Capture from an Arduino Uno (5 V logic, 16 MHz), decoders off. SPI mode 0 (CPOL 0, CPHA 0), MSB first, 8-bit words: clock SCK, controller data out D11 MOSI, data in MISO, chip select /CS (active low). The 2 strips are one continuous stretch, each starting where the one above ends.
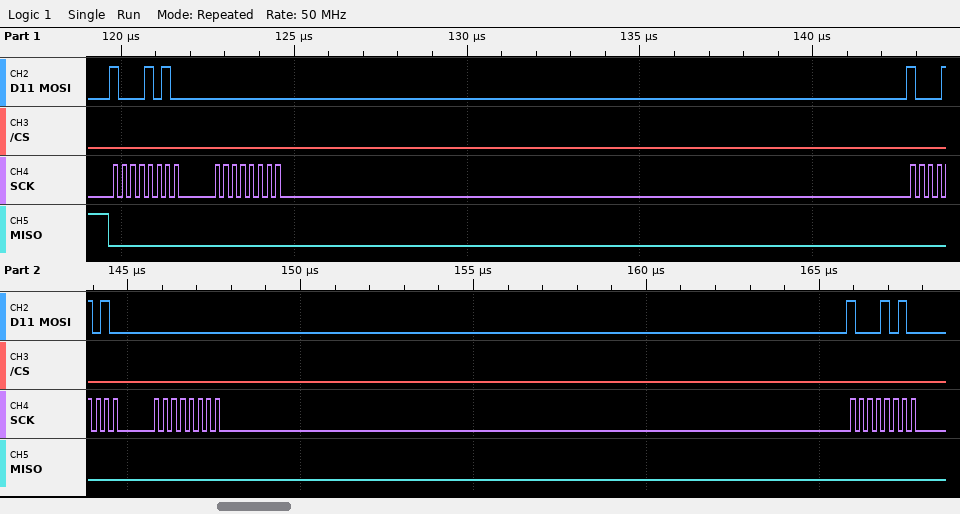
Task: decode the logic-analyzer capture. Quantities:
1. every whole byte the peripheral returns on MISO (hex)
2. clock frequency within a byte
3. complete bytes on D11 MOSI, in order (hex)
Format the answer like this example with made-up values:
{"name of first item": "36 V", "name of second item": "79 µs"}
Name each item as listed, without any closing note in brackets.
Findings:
{"every whole byte the peripheral returns on MISO": "00 00 00 00 00", "clock frequency within a byte": "4 MHz", "complete bytes on D11 MOSI, in order": "8A 00 8A 00 8A"}
